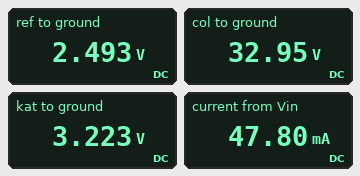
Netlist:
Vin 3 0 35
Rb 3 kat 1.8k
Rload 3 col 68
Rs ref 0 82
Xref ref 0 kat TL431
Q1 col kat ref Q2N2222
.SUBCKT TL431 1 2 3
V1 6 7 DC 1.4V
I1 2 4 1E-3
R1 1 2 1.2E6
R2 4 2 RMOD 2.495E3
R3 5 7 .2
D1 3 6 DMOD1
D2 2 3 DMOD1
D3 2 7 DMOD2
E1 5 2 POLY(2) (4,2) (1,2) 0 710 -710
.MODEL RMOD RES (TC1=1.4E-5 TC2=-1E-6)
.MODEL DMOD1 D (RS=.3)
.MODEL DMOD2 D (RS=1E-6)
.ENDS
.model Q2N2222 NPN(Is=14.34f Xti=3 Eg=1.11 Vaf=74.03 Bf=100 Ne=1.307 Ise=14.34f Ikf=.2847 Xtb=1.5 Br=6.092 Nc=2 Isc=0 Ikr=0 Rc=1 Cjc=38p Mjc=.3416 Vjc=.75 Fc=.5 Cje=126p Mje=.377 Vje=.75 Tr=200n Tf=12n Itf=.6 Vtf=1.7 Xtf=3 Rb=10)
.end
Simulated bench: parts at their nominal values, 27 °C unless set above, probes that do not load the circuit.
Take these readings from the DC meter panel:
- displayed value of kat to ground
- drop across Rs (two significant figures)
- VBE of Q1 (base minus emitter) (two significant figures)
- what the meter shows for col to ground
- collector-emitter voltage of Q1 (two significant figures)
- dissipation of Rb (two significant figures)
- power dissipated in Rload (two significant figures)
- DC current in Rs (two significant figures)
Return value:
3.223 V
2.5 V
730 mV
32.95 V
30 V
560 mW
62 mW
30 mA
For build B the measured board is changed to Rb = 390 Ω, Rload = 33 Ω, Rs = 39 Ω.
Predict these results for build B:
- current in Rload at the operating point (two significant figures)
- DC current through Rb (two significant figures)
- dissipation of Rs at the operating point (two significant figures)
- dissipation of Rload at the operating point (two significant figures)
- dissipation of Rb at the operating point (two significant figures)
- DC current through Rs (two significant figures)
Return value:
63 mA
81 mA
160 mW
130 mW
2.6 W
64 mA
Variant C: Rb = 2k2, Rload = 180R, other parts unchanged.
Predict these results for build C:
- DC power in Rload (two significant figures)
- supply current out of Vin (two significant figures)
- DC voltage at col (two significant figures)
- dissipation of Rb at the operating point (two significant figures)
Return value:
160 mW
45 mA
30 V
460 mW
